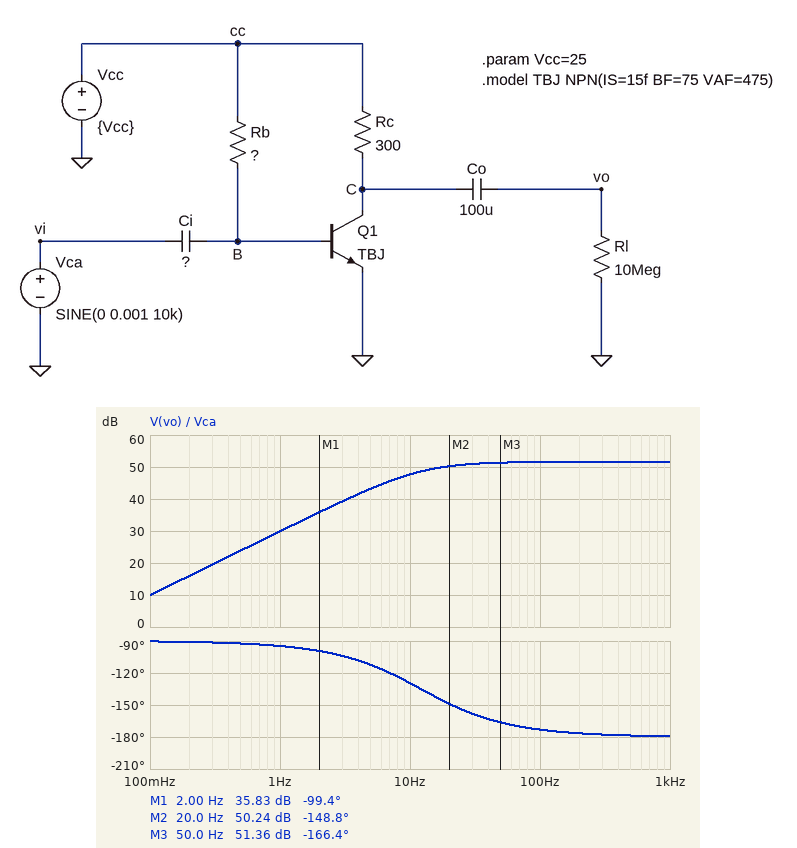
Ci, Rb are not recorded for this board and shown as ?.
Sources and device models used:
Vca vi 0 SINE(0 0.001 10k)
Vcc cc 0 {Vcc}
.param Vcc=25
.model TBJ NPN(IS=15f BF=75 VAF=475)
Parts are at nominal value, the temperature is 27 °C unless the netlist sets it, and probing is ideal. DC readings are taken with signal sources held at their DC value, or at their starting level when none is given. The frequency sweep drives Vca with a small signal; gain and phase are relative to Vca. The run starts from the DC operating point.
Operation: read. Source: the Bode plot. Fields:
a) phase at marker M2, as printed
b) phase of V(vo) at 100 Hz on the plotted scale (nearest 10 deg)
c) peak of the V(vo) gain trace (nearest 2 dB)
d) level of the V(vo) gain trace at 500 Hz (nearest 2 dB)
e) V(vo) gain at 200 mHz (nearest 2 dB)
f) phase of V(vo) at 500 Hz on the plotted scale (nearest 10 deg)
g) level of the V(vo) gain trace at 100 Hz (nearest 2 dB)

-148.8 deg
-170 deg
52 dB
52 dB
16 dB
-180 deg
52 dB
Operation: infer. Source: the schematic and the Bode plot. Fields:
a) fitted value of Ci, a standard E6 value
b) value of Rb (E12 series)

220 µF
56 kΩ
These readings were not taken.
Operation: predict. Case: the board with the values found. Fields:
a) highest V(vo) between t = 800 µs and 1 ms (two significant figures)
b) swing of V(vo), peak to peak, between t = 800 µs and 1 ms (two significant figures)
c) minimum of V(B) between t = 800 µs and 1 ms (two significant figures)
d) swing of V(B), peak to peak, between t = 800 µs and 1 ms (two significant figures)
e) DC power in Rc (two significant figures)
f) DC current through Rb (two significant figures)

370 mV
760 mV
730 mV
2.0 mV
340 mW
430 µA
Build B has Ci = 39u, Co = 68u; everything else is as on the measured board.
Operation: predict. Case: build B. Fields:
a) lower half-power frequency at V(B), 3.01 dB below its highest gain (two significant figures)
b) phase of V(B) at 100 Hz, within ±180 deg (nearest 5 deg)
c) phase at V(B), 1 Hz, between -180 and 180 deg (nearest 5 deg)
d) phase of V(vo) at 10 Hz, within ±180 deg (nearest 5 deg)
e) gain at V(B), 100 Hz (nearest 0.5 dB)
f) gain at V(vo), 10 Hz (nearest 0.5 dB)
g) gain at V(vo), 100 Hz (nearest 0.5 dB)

68 Hz
35 deg
90 deg
-100 deg
-1.5 dB
35.0 dB
50.0 dB
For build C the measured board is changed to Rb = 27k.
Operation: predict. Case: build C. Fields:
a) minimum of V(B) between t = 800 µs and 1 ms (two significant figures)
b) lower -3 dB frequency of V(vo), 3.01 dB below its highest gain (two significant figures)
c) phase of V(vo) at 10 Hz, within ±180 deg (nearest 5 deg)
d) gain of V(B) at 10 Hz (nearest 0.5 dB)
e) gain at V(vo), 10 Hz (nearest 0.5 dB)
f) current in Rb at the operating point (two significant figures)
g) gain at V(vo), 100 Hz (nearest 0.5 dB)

750 mV
25 Hz
-110 deg
-8.5 dB
49.0 dB
900 µA
57.5 dB
